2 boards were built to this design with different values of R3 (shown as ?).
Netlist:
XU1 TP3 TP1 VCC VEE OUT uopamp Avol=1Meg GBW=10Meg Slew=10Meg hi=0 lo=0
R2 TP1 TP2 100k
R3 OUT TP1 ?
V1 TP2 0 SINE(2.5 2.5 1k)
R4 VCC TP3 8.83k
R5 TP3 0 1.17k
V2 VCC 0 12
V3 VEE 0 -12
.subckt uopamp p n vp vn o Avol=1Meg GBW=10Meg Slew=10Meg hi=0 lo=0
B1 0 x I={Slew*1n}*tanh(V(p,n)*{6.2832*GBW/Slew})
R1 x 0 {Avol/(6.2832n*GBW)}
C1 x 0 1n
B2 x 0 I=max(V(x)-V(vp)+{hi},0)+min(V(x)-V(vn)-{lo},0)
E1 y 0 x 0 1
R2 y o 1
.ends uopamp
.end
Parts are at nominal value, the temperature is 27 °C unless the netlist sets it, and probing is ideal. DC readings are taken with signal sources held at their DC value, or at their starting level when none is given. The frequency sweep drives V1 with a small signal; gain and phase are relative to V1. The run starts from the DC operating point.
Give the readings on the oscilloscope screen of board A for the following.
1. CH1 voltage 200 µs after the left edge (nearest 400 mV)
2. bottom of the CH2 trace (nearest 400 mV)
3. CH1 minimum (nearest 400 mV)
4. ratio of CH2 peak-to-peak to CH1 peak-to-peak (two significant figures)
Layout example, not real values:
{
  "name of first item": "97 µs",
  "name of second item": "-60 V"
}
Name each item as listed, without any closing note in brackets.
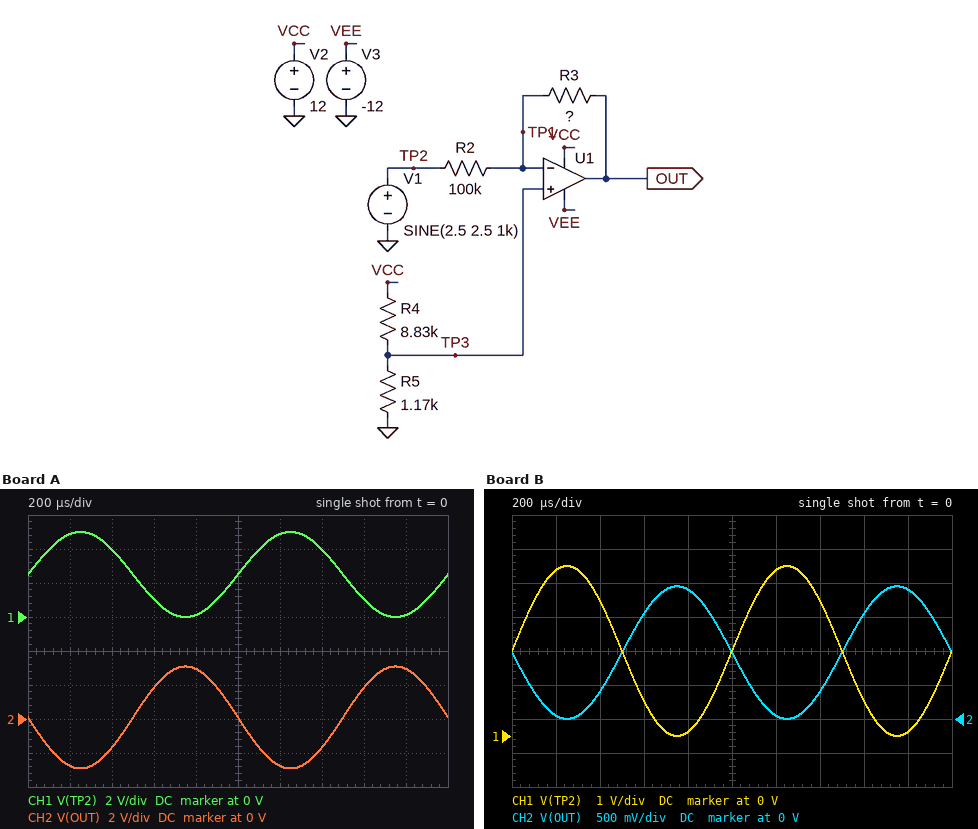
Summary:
{
  "CH1 voltage 200 µs after the left edge": "4.8 V",
  "bottom of the CH2 trace": "-2.8 V",
  "CH1 minimum": "0 V",
  "ratio of CH2 peak-to-peak to CH1 peak-to-peak": "1.2"
}
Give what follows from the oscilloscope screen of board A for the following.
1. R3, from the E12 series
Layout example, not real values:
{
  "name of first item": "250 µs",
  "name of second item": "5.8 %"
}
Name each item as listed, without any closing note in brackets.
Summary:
{
  "R3, from the E12 series": "120 kΩ"
}
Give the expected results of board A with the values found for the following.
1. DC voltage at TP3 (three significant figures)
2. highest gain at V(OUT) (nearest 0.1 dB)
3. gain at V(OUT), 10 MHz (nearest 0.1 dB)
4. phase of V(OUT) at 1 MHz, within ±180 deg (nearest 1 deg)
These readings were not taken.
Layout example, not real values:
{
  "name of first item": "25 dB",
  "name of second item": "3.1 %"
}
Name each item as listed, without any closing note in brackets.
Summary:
{
  "DC voltage at TP3": "1.40 V",
  "highest gain at V(OUT)": "1.6 dB",
  "gain at V(OUT), 10 MHz": "-6.1 dB",
  "phase of V(OUT) at 1 MHz, within ±180 deg": "168 deg"
}
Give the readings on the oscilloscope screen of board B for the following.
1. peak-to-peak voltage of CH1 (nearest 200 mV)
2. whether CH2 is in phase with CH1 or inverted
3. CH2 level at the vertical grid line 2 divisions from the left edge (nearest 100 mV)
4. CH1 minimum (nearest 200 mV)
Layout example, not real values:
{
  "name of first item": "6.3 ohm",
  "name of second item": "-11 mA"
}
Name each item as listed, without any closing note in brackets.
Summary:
{
  "peak-to-peak voltage of CH1": "5.0 V",
  "whether CH2 is in phase with CH1 or inverted": "inverted",
  "CH2 level at the vertical grid line 2 divisions from the left edge": "400 mV",
  "CH1 minimum": "0 V"
}
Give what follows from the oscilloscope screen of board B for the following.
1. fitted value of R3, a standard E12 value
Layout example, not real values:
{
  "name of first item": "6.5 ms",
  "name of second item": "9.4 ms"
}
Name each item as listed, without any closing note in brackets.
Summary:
{
  "fitted value of R3, a standard E12 value": "39 kΩ"
}
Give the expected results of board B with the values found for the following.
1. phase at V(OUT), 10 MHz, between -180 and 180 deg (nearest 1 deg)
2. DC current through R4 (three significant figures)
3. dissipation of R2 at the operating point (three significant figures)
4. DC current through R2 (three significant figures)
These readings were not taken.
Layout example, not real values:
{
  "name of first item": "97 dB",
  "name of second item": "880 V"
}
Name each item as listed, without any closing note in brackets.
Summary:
{
  "phase at V(OUT), 10 MHz, between -180 and 180 deg": "126 deg",
  "DC current through R4": "1.20 mA",
  "dissipation of R2 at the operating point": "12.0 µW",
  "DC current through R2": "11.0 µA"
}
